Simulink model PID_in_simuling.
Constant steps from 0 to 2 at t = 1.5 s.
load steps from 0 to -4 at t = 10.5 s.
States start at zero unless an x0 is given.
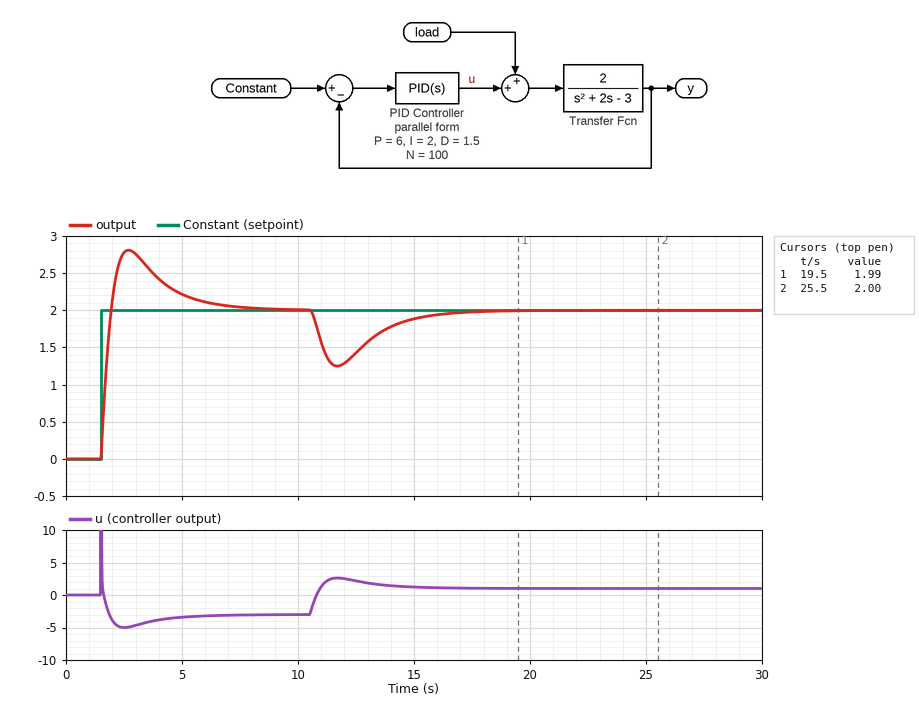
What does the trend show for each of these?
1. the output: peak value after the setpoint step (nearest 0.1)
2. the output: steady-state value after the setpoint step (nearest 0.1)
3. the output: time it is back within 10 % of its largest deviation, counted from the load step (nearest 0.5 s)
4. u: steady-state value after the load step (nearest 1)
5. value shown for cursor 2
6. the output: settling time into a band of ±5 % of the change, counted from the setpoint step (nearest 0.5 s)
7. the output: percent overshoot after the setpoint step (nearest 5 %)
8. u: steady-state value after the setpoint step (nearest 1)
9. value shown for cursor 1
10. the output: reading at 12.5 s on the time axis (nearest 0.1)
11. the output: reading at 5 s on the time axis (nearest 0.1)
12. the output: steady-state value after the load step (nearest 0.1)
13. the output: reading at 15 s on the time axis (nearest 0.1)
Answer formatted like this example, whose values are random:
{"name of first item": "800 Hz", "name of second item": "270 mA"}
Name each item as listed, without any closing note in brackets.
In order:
{"the output: peak value after the setpoint step": "2.8", "the output: steady-state value after the setpoint step": "2.0", "the output: time it is back within 10 % of its largest deviation, counted from the load step": "5.0 s", "u: steady-state value after the load step": "1", "value shown for cursor 2": "2.00", "the output: settling time into a band of ±5 % of the change, counted from the setpoint step": "4.5 s", "the output: percent overshoot after the setpoint step": "40 %", "u: steady-state value after the setpoint step": "-3", "value shown for cursor 1": "1.99", "the output: reading at 12.5 s on the time axis": "1.4", "the output: reading at 5 s on the time axis": "2.2", "the output: steady-state value after the load step": "2.0", "the output: reading at 15 s on the time axis": "1.9"}
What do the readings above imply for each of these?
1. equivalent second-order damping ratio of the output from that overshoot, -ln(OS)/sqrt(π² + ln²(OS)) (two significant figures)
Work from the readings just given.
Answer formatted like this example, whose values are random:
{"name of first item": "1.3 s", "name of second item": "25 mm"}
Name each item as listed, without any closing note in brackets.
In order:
{"equivalent second-order damping ratio of the output from that overshoot, -ln(OS)/sqrt(π² + ln²(OS))": "0.28"}
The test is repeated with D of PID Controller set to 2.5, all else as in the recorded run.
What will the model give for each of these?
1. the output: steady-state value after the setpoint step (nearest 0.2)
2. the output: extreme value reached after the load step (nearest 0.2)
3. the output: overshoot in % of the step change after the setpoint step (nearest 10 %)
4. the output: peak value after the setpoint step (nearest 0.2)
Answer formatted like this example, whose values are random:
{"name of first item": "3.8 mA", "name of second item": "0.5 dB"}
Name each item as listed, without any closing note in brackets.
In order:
{"the output: steady-state value after the setpoint step": "2.0", "the output: extreme value reached after the load step": "1.4", "the output: overshoot in % of the step change after the setpoint step": "30 %", "the output: peak value after the setpoint step": "2.6"}
